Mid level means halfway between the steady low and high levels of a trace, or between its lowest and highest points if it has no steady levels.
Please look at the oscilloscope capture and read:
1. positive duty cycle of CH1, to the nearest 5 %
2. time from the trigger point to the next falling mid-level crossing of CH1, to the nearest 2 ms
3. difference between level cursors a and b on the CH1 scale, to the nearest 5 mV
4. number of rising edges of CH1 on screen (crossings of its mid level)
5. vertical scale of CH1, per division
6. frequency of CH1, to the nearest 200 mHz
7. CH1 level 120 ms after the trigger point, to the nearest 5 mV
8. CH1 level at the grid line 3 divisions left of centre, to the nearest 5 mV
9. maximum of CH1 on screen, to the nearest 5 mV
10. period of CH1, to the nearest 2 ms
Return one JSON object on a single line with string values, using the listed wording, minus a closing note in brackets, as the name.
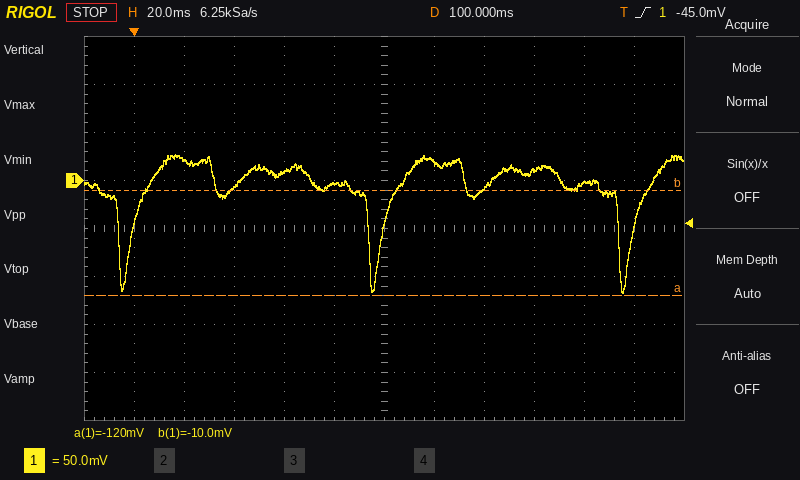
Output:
{"positive duty cycle of CH1, to the nearest 5 %": "95 %", "time from the trigger point to the next falling mid-level crossing of CH1, to the nearest 2 ms": "94 ms", "difference between level cursors a and b on the CH1 scale, to the nearest 5 mV": "110 mV", "number of rising edges of CH1 on screen": "3", "vertical scale of CH1, per division": "50 mV", "frequency of CH1, to the nearest 200 mHz": "10.0 Hz", "CH1 level 120 ms after the trigger point, to the nearest 5 mV": "20 mV", "CH1 level at the grid line 3 divisions left of centre, to the nearest 5 mV": "-5 mV", "maximum of CH1 on screen, to the nearest 5 mV": "25 mV", "period of CH1, to the nearest 2 ms": "100 ms"}
